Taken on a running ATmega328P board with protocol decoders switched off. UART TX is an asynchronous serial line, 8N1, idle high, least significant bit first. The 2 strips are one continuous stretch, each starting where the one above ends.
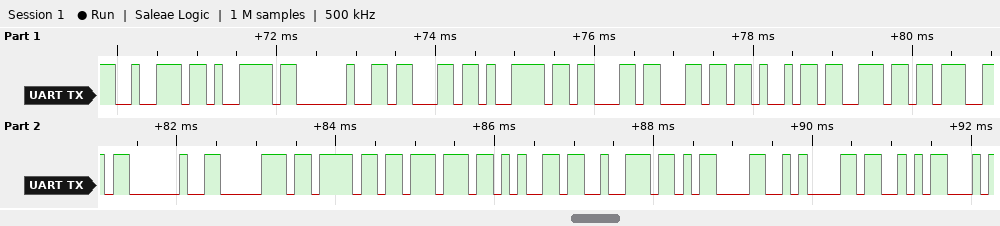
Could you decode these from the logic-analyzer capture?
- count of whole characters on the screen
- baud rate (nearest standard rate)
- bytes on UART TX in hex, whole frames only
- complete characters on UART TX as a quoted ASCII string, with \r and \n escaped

19
9600 baud
72 79 20 63 79 63 6C 69 6E 67 20 70 6F 77 65 72 0D 0A 53
"ry cycling power\r\nS"
